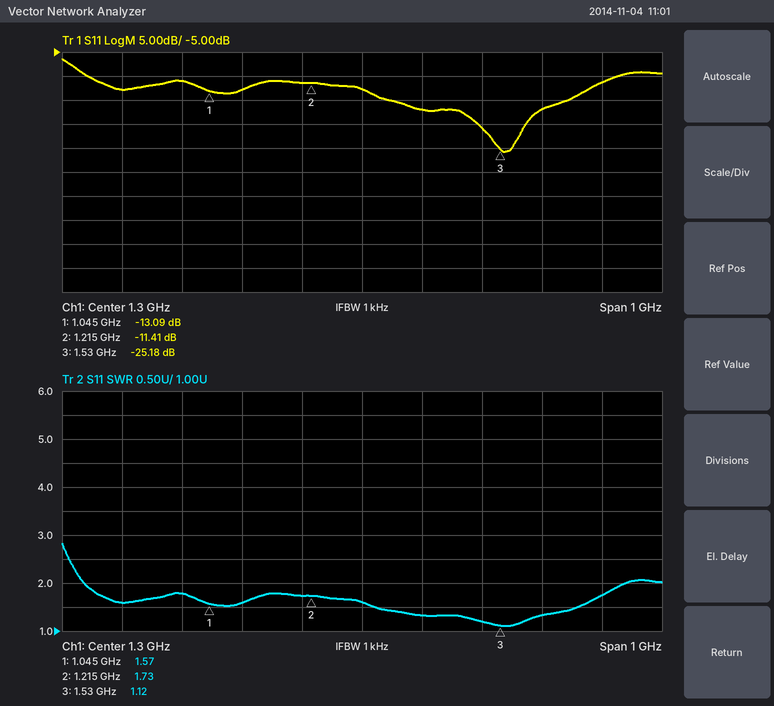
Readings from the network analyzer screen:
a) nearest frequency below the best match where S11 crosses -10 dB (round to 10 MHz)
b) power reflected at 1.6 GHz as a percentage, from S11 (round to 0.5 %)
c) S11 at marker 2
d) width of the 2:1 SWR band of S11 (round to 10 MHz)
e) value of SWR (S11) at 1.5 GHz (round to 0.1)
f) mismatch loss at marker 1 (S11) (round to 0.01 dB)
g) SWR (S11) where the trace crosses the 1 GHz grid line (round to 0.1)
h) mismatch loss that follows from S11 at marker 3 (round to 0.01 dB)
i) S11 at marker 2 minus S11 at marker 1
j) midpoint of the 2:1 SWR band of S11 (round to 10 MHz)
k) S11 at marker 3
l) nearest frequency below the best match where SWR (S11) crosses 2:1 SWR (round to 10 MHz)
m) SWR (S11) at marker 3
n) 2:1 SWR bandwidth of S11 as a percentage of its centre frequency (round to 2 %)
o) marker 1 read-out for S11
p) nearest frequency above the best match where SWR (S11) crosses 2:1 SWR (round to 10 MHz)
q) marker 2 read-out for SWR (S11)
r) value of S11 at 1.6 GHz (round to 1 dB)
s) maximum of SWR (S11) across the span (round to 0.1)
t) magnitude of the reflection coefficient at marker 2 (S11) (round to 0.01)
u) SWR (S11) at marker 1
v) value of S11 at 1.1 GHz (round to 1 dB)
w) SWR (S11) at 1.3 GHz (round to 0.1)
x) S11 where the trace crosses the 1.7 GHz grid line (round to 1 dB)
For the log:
840 MHz
2.0 %
-11.41 dB
900 MHz
1.2
0.22 dB
1.8
0.01 dB
1.68 dB
1.29 GHz
-25.18 dB
840 MHz
1.12
70 %
-13.09 dB
1.74 GHz
1.73
-17 dB
2.8
0.27
1.57
-13 dB
1.6
-11 dB
